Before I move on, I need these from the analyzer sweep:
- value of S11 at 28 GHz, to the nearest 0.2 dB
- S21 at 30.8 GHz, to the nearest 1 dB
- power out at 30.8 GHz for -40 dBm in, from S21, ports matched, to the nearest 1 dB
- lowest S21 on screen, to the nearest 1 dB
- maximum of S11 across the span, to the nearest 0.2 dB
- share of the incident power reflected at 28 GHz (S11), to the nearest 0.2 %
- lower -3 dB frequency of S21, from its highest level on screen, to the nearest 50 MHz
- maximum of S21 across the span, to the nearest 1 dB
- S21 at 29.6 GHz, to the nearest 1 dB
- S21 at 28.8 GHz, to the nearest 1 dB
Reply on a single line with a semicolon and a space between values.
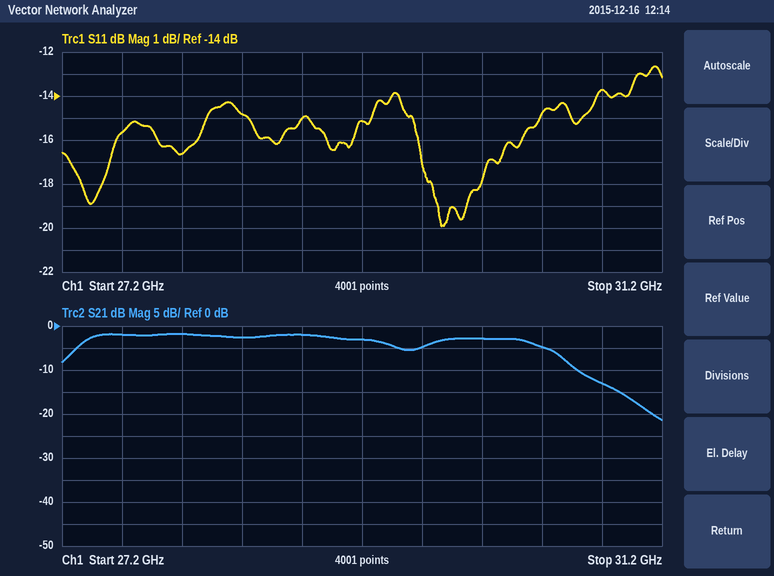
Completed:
-16.6 dB; -13 dB; -53 dBm; -21 dB; -12.6 dB; 2.2 %; 27.30 GHz; -2 dB; -5 dB; -2 dB
